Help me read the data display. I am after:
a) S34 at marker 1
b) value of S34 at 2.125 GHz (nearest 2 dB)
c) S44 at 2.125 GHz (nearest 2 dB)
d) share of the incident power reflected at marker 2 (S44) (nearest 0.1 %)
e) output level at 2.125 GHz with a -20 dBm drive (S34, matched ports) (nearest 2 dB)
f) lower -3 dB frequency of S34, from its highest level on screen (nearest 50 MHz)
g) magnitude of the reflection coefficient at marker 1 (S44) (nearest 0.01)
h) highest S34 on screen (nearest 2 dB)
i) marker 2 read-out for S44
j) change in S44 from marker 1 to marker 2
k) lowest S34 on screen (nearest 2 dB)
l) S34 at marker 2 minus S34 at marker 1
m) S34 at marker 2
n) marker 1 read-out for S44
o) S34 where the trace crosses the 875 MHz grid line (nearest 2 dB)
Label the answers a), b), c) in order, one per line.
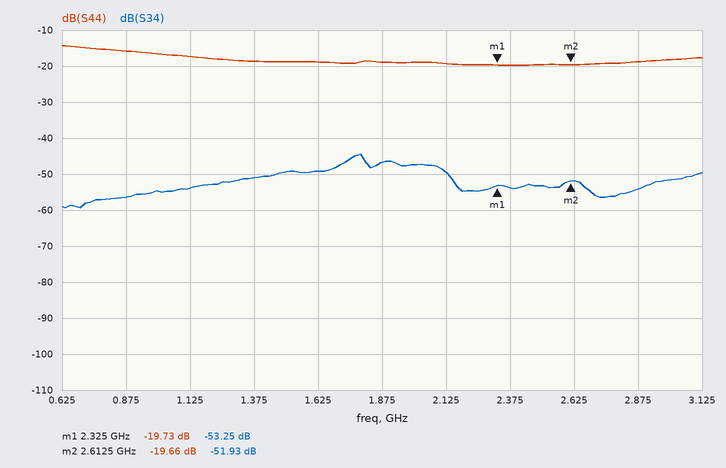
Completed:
a) -53.25 dB
b) -50 dB
c) -20 dB
d) 1.1 %
e) -70 dBm
f) 1.70 GHz
g) 0.10
h) -44 dB
i) -19.66 dB
j) 0.07 dB
k) -60 dB
l) 1.32 dB
m) -51.93 dB
n) -19.73 dB
o) -56 dB
